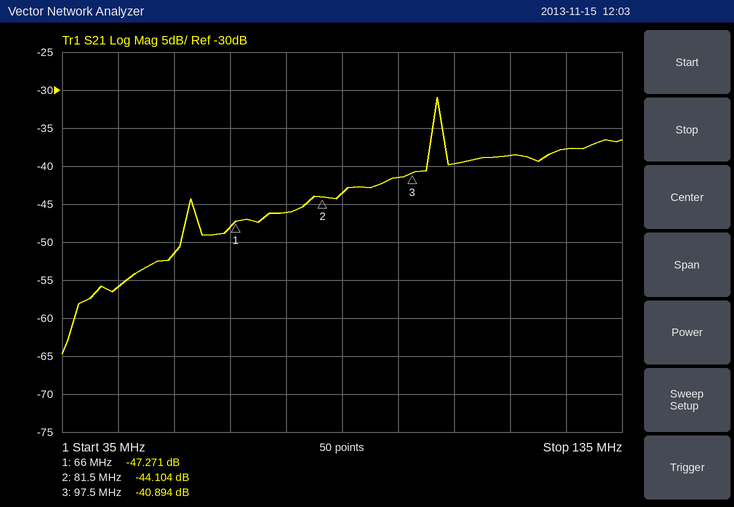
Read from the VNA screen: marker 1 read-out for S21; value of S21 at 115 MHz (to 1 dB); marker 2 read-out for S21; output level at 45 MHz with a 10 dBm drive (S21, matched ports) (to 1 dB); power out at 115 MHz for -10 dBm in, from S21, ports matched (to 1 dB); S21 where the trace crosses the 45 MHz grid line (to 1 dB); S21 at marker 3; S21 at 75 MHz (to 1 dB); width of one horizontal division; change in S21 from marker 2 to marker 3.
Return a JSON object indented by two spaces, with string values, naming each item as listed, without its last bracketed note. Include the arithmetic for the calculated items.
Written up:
{
  "marker 1 read-out for S21": "-47.271 dB",
  "value of S21 at 115 MHz": "-39 dB",
  "marker 2 read-out for S21": "-44.104 dB",
  "output level at 45 MHz with a 10 dBm drive (S21, matched ports)": "10 dBm + (-56 dB) = -46 dBm",
  "power out at 115 MHz for -10 dBm in, from S21, ports matched": "-10 dBm + (-39 dB) = -49 dBm",
  "S21 where the trace crosses the 45 MHz grid line": "-56 dB",
  "S21 at marker 3": "-40.894 dB",
  "S21 at 75 MHz": "-46 dB",
  "width of one horizontal division": "10 MHz",
  "change in S21 from marker 2 to marker 3": "-40.894 − (-44.104) = 3.210 dB"
}
